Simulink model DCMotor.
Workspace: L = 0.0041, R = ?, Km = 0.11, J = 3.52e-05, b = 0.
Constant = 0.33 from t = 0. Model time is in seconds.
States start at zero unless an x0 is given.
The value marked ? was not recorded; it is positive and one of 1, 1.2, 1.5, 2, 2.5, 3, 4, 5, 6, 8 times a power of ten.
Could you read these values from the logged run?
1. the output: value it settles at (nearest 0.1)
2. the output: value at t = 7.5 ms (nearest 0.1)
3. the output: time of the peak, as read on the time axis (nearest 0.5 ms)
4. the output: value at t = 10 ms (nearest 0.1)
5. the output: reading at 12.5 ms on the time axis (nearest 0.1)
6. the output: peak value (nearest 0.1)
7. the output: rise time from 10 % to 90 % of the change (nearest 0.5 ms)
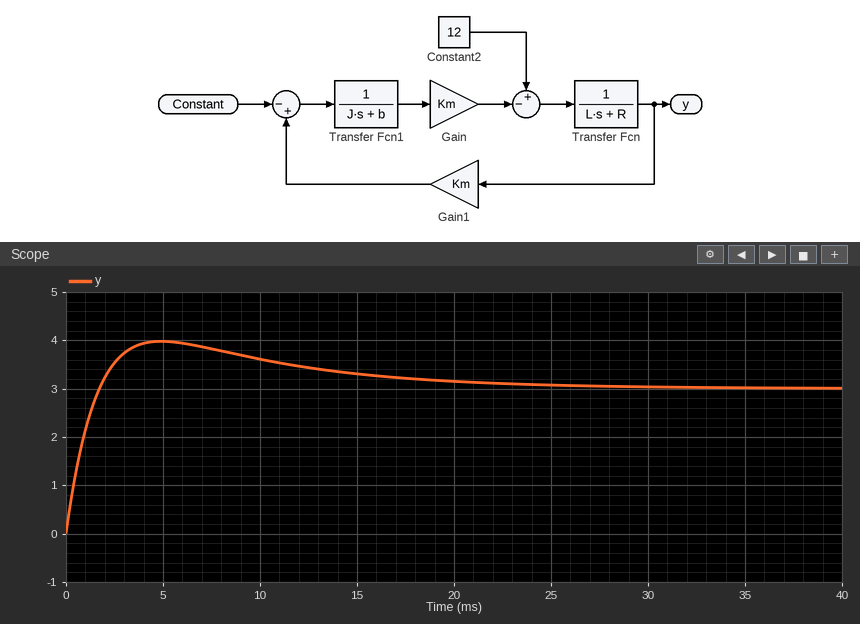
3.0
3.8
5.0 ms
3.6
3.4
4.0
1.5 ms
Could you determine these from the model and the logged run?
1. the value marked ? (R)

3
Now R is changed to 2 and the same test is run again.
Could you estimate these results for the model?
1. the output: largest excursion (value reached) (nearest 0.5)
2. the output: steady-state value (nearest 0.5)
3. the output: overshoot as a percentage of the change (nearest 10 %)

5.5
3.0
80 %
